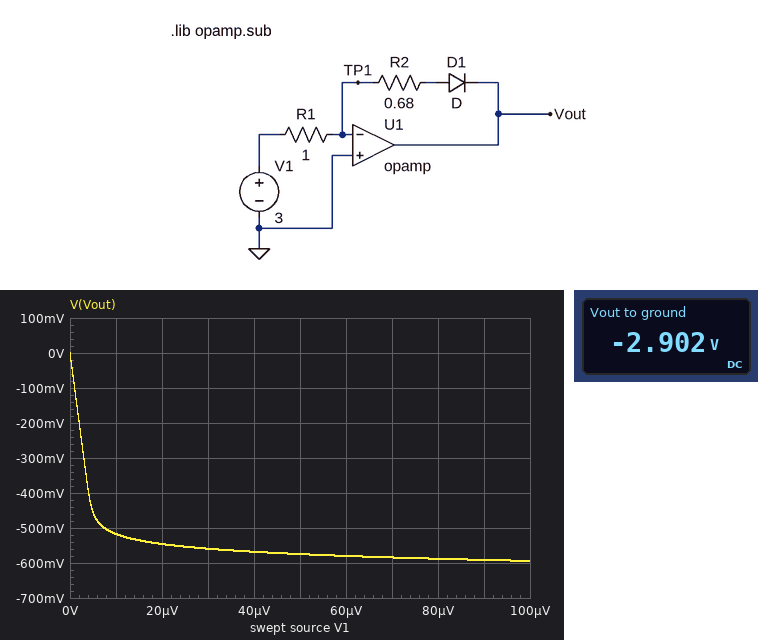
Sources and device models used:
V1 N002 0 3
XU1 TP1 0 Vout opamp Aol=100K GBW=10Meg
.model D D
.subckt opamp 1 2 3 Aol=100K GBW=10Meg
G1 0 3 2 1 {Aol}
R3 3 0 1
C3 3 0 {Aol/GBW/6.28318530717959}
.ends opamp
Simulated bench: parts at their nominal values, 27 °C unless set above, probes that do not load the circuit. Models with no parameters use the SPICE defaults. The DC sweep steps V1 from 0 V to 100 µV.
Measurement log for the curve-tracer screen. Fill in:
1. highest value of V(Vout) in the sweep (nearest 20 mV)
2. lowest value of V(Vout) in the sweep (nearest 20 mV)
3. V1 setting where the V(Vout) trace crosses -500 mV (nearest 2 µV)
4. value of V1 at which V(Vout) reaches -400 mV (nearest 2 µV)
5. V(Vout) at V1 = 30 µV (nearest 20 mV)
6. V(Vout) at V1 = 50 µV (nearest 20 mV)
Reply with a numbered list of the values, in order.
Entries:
1. 0 V
2. -600 mV
3. 8 µV
4. 4 µV
5. -560 mV
6. -580 mV
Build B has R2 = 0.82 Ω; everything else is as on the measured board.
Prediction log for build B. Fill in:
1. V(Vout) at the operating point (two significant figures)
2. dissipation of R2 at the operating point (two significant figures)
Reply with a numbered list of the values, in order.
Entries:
1. -3.3 V
2. 7.4 W
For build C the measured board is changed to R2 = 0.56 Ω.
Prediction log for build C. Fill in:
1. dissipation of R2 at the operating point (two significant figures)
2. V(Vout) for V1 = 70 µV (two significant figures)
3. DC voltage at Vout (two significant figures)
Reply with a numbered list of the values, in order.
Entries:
1. 5.0 W
2. -580 mV
3. -2.5 V
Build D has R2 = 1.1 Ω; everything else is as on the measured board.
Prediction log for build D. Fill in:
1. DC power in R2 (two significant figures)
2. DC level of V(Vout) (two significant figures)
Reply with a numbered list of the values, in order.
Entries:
1. 9.9 W
2. -4.2 V
